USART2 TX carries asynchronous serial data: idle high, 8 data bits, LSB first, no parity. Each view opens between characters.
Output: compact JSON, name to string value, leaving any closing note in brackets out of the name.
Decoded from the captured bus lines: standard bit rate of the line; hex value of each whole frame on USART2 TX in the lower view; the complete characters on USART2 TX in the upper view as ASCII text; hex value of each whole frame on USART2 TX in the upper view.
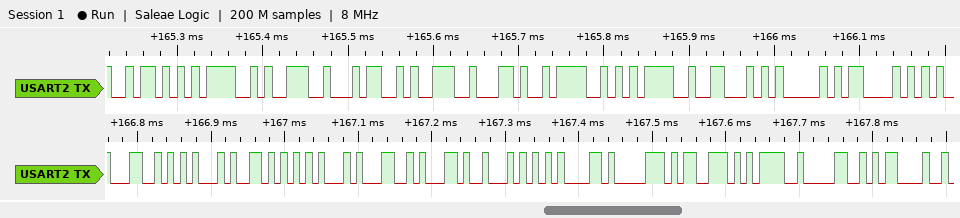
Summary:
{"standard bit rate of the line": "115200 baud", "hex value of each whole frame on USART2 TX in the lower view": "4C, 45, 56, 45, 4C, 2C, 54, 61, 70, 73, 3D, 30, 0D", "the complete characters on USART2 TX in the upper view as ASCII text": "\"Z=949,O=FAC\"", "hex value of each whole frame on USART2 TX in the upper view": "5A, 3D, 39, 34, 39, 2C, 4F, 3D, 46, 41, 43"}
